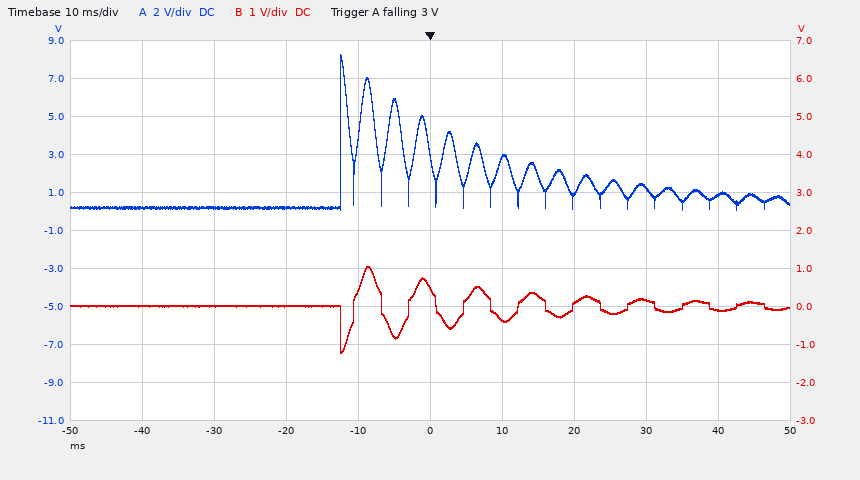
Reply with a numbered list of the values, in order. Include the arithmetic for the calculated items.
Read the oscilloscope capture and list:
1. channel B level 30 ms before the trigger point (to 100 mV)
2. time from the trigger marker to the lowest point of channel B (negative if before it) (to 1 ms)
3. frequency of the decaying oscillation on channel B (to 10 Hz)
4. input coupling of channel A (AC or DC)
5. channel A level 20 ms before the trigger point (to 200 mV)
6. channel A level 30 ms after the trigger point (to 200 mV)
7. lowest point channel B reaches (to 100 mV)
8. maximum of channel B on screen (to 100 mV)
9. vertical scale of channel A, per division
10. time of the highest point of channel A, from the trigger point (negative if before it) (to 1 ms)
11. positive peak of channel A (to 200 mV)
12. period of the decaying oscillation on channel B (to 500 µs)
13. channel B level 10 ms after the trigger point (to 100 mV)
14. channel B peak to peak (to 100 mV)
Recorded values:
1. 0.0 V
2. -12 ms
3. 1 / 7.5 ms ≈ 133 Hz, so 130 Hz to the nearest 10 Hz
4. DC
5. 200 mV
6. 1.2 V
7. -1.2 V
8. 1.1 V
9. 2 V
10. -12 ms
11. 8.2 V
12. 7.5 ms
13. -300 mV
14. 1.1 V − (-1.2 V) = 2.3 V
